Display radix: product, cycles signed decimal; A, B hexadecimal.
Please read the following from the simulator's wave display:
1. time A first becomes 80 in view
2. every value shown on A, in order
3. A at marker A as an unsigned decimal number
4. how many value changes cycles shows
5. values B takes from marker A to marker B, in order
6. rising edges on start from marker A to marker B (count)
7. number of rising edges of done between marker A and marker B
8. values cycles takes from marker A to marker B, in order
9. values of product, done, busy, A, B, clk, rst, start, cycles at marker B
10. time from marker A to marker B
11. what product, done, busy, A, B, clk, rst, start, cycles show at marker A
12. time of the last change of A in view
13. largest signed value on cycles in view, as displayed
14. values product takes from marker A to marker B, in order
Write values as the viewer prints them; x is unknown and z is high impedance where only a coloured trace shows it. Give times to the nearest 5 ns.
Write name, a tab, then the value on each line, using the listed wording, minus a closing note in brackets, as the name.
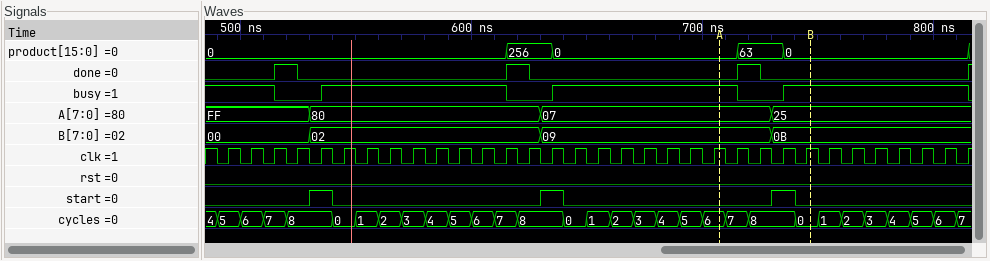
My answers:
time A first becomes 80 in view	530 ns
every value shown on A, in order	FF, 80, 07, 25
A at marker A as an unsigned decimal number	7
how many value changes cycles shows	30
values B takes from marker A to marker B, in order	09, 0B
rising edges on start from marker A to marker B	1
number of rising edges of done between marker A and marker B	1
values cycles takes from marker A to marker B, in order	6, 7, 8, 0
values of product, done, busy, A, B, clk, rst, start, cycles at marker B	product=0, done=0, busy=1, A=25, B=0B, clk=1, rst=0, start=0, cycles=0
time from marker A to marker B	40 ns
what product, done, busy, A, B, clk, rst, start, cycles show at marker A	product=0, done=0, busy=1, A=07, B=09, clk=1, rst=0, start=0, cycles=6
time of the last change of A in view	730 ns
largest signed value on cycles in view, as displayed	8
values product takes from marker A to marker B, in order	0, 63, 0
